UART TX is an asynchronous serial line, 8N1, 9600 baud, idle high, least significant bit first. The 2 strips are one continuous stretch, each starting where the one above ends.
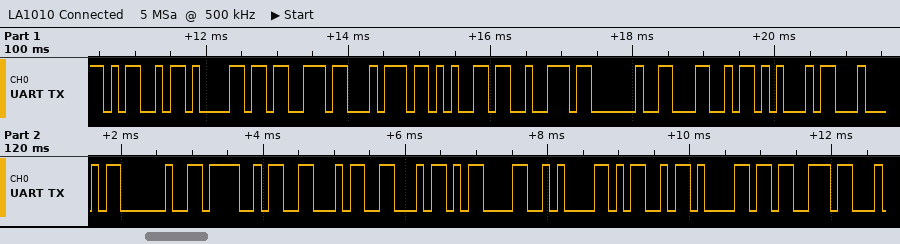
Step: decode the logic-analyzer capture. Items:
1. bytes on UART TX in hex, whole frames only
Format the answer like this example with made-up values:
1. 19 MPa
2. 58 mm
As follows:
1. 4D 61 73 74 65 72 20 4C 45 44 20 4F 46 46 0D 0A 4D 61 73
